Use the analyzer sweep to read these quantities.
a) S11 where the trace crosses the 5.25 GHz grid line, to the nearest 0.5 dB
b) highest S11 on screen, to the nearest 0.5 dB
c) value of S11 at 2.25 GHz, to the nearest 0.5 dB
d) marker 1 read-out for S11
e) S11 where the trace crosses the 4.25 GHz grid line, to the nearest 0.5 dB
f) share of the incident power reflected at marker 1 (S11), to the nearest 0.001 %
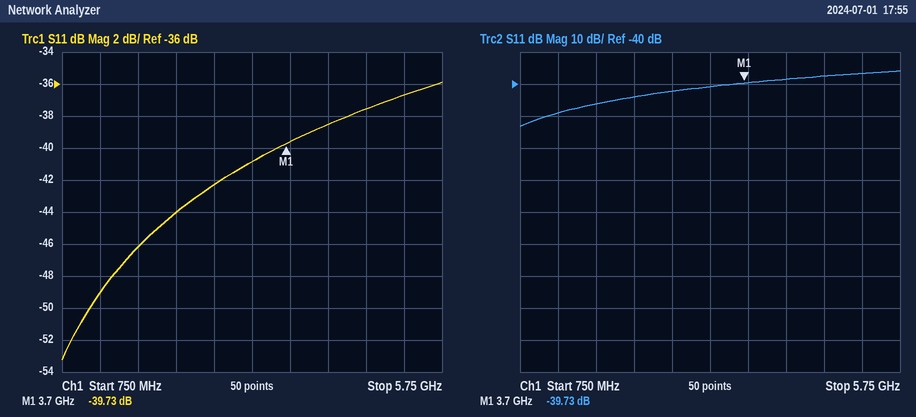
-36.5 dB
-36.0 dB
-44.0 dB
-39.73 dB
-38.5 dB
0.011 %
